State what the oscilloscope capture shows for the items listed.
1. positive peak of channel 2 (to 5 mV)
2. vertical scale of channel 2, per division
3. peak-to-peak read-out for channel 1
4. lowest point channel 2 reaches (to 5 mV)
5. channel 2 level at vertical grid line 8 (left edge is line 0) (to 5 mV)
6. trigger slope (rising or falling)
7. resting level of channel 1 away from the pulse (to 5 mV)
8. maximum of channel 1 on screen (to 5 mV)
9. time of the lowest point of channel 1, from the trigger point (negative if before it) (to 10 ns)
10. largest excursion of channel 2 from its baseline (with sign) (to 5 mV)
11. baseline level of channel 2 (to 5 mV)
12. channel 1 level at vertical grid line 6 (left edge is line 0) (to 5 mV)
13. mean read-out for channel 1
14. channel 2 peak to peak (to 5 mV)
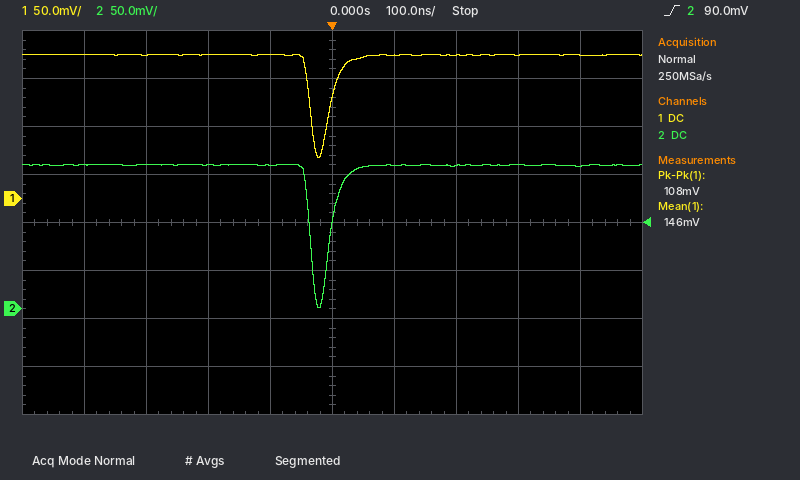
150 mV
50 mV
108 mV
0 mV
150 mV
rising
150 mV
150 mV
-20 ns
-150 mV
150 mV
150 mV
146 mV
150 mV
